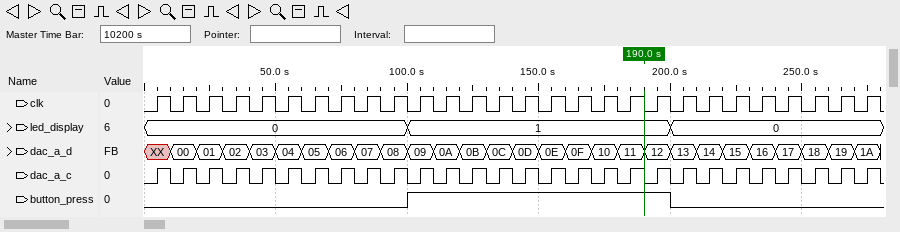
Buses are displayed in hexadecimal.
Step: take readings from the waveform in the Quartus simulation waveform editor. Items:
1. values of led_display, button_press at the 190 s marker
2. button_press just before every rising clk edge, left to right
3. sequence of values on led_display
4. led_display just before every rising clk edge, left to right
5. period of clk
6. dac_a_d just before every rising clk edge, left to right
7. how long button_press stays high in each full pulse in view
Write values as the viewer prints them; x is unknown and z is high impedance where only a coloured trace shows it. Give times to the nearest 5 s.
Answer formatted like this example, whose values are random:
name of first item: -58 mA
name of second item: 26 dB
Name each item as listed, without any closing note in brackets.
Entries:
values of led_display, button_press at the 190 s marker: led_display=1, button_press=1
button_press just before every rising clk edge, left to right: 0 0 0 0 0 0 0 0 0 0 1 1 1 1 1 1 1 1 1 1 0 0 0 0 0 0 0 0
sequence of values on led_display: 0, 1, 0
led_display just before every rising clk edge, left to right: 0, 0, 0, 0, 0, 0, 0, 0, 0, 0, 1, 1, 1, 1, 1, 1, 1, 1, 1, 1, 0, 0, 0, 0, 0, 0, 0, 0
period of clk: 10 s
dac_a_d just before every rising clk edge, left to right: XX, 00, 01, 02, 03, 04, 05, 06, 07, 08, 09, 0A, 0B, 0C, 0D, 0E, 0F, 10, 11, 12, 13, 14, 15, 16, 17, 18, 19, 1A
how long button_press stays high in each full pulse in view: 100 s
